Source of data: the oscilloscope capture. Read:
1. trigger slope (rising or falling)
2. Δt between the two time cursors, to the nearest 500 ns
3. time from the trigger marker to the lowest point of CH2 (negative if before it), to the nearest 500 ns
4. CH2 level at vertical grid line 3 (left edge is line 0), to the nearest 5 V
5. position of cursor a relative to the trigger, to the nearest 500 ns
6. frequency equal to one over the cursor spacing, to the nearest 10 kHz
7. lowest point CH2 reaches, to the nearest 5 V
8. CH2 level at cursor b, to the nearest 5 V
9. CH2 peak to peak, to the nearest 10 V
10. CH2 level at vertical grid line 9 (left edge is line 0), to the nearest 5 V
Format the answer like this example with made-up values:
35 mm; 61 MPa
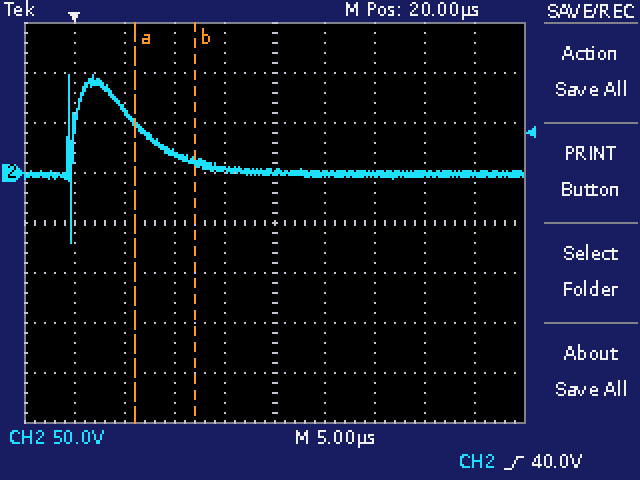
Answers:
rising; 6.0 µs; -500 ns; 20 V; +6.0 µs; 170 kHz; -70 V; 10 V; 170 V; 0 V
